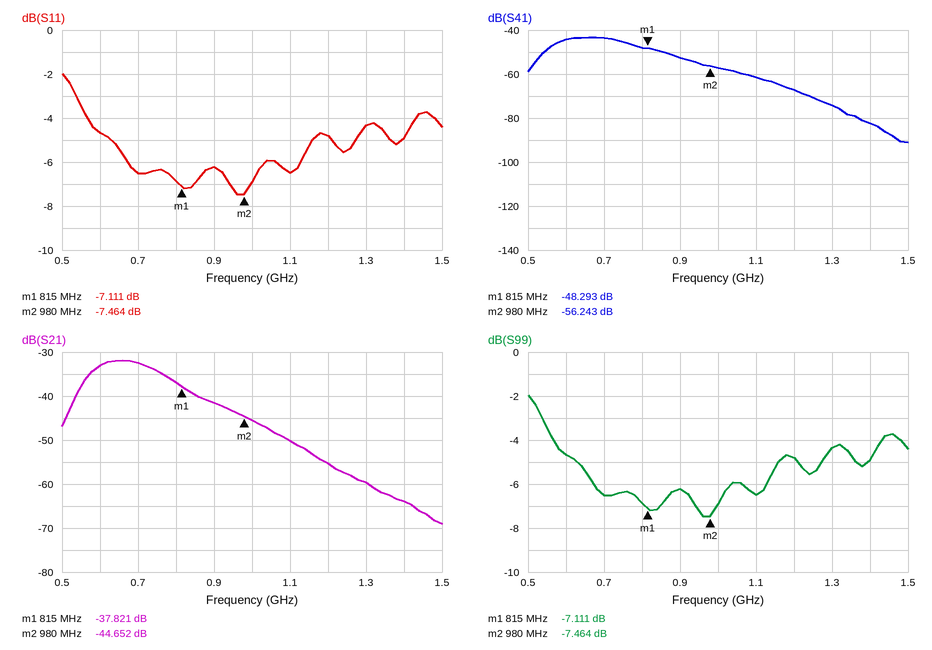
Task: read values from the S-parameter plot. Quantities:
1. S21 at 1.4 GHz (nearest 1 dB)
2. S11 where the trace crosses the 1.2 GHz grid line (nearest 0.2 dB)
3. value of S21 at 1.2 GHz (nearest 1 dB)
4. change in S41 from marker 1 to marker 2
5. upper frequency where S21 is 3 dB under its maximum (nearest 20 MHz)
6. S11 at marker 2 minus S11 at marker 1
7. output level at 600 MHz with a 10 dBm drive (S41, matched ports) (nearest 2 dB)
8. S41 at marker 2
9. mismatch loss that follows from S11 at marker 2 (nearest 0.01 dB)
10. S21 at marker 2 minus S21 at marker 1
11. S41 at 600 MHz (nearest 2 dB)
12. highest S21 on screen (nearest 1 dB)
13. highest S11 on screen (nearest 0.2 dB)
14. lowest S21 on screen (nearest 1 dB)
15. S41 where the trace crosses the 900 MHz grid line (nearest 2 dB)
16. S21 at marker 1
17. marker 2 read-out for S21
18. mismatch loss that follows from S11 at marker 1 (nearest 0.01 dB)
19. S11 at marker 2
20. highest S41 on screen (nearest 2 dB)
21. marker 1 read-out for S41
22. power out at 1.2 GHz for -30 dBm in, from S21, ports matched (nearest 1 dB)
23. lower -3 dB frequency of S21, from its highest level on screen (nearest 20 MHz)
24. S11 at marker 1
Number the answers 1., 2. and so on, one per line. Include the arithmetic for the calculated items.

1. -64 dB
2. -4.8 dB
3. -55 dB
4. -56.243 − (-48.293) = -7.950 dB
5. 760 MHz
6. -7.464 − (-7.111) = -0.353 dB
7. 10 dBm + (-44 dB) = -34 dBm
8. -56.243 dB
9. −10 log10(1 − 10^(-7.464/10)) ≈ 0.86 dB
10. -44.652 − (-37.821) = -6.831 dB
11. -44 dB
12. -32 dB
13. -2.0 dB
14. -69 dB
15. -52 dB
16. -37.821 dB
17. -44.652 dB
18. −10 log10(1 − 10^(-7.111/10)) ≈ 0.94 dB
19. -7.464 dB
20. -44 dB
21. -48.293 dB
22. -30 dBm + (-55 dB) = -85 dBm
23. 580 MHz
24. -7.111 dB
